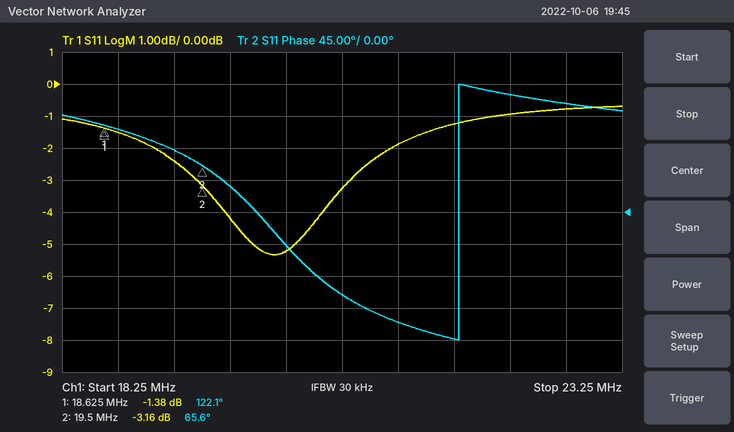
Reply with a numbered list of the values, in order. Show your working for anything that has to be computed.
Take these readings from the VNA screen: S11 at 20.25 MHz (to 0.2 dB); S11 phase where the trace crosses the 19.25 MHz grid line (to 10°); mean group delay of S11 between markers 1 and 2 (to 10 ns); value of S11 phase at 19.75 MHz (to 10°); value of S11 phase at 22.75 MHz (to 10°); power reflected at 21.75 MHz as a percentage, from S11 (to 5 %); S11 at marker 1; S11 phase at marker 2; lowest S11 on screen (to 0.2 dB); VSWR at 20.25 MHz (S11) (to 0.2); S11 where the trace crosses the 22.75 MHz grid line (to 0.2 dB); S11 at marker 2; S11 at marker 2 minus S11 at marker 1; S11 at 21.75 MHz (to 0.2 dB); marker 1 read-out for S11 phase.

1. -5.2 dB
2. 90°
3. −(65.6° − (122.1°))/(360° × 875 kHz) ≈ 179 ns, so 180 ns to the nearest 10 ns
4. 40°
5. 150°
6. 10^(-1.2/10) ≈ 75.9 %, so 75 % to the nearest 5 %
7. -1.38 dB
8. 65.6°
9. -5.4 dB
10. |Γ| = 10^(-5.2/20) = 0.5495; VSWR = (1 + 0.5495)/(1 − 0.5495) ≈ 3.4
11. -0.8 dB
12. -3.16 dB
13. -3.16 − (-1.38) = -1.78 dB
14. -1.2 dB
15. 122.1°
